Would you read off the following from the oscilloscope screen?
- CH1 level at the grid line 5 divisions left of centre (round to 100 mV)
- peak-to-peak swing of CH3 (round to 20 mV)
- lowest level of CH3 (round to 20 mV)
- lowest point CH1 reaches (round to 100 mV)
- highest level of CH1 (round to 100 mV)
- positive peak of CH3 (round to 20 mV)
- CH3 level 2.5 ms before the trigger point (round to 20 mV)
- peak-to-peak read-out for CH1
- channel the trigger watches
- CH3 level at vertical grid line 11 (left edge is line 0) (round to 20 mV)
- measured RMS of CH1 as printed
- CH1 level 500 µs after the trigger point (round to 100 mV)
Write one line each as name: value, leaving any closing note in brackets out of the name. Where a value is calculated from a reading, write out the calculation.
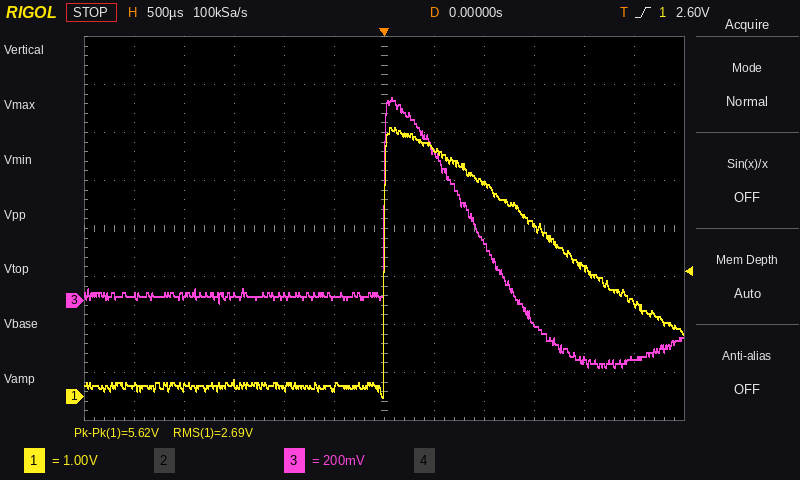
CH1 level at the grid line 5 divisions left of centre: 200 mV
peak-to-peak swing of CH3: 840 mV − (-280 mV) = 1.12 V
lowest level of CH3: -280 mV
lowest point CH1 reaches: 0.0 V
highest level of CH1: 5.6 V
positive peak of CH3: 840 mV
CH3 level 2.5 ms before the trigger point: 20 mV
peak-to-peak read-out for CH1: 5.62 V
channel the trigger watches: CH1
CH3 level at vertical grid line 11 (left edge is line 0): -240 mV
measured RMS of CH1 as printed: 2.69 V
CH1 level 500 µs after the trigger point: 5.2 V
